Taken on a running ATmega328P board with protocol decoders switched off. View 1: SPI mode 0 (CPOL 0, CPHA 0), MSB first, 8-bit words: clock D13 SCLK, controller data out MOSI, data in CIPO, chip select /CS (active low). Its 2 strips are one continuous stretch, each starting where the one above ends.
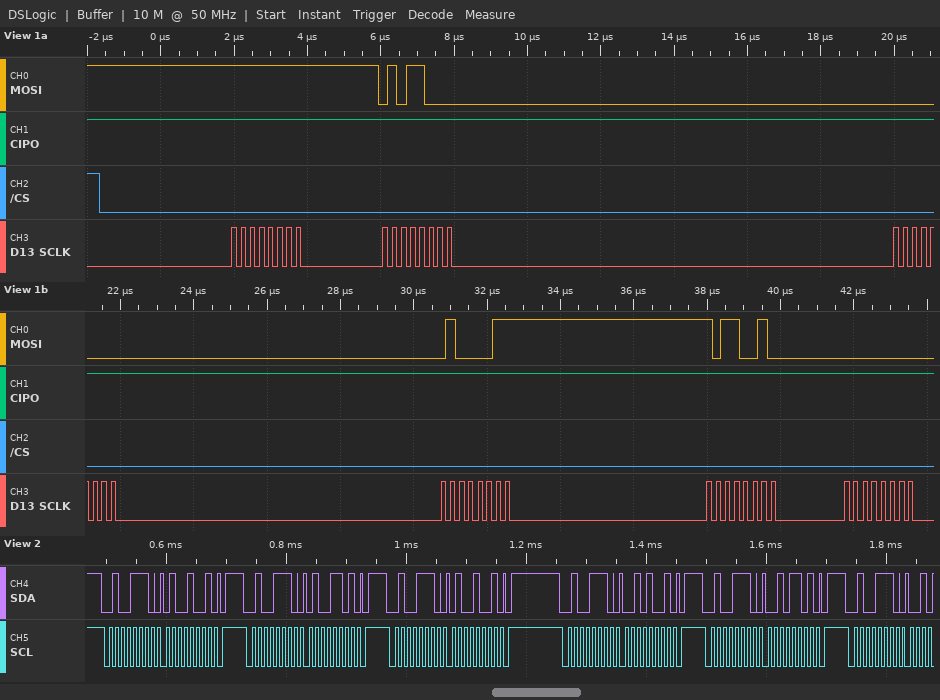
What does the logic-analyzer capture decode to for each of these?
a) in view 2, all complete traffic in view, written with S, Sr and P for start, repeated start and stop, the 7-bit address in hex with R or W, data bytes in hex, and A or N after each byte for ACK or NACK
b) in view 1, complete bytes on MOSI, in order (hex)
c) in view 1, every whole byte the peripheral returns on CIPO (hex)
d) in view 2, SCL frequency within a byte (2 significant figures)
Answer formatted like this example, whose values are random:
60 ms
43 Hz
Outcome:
S 27W A 49 A P S 27W A 4D A P S 27W A 49 A P S 27W A 29 A P S 27W A 2D A P S 27W A
0xFF 0x58 0x00 0x43 0xB2 0x00
0xFF 0xFF 0xFF 0xFF 0xFF 0xFF
100 kHz
